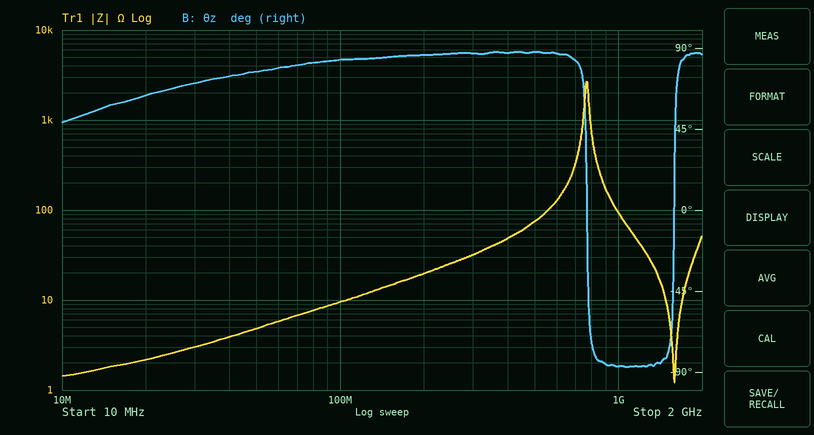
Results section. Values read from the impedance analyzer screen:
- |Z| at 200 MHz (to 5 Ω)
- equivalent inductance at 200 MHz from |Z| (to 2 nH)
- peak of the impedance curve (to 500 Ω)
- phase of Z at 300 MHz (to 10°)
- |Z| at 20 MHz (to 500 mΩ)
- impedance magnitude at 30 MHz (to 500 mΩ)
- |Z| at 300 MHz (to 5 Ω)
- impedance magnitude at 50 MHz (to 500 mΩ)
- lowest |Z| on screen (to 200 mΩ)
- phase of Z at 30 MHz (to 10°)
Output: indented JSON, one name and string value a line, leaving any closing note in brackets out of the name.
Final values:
{
  "|Z| at 200 MHz": "20 Ω",
  "equivalent inductance at 200 MHz from |Z|": "16 nH",
  "peak of the impedance curve": "2.5 kΩ",
  "phase of Z at 300 MHz": "90°",
  "|Z| at 20 MHz": "2.0 Ω",
  "impedance magnitude at 30 MHz": "3.0 Ω",
  "|Z| at 300 MHz": "30 Ω",
  "impedance magnitude at 50 MHz": "5.0 Ω",
  "lowest |Z| on screen": "1.2 Ω",
  "phase of Z at 30 MHz": "70°"
}
